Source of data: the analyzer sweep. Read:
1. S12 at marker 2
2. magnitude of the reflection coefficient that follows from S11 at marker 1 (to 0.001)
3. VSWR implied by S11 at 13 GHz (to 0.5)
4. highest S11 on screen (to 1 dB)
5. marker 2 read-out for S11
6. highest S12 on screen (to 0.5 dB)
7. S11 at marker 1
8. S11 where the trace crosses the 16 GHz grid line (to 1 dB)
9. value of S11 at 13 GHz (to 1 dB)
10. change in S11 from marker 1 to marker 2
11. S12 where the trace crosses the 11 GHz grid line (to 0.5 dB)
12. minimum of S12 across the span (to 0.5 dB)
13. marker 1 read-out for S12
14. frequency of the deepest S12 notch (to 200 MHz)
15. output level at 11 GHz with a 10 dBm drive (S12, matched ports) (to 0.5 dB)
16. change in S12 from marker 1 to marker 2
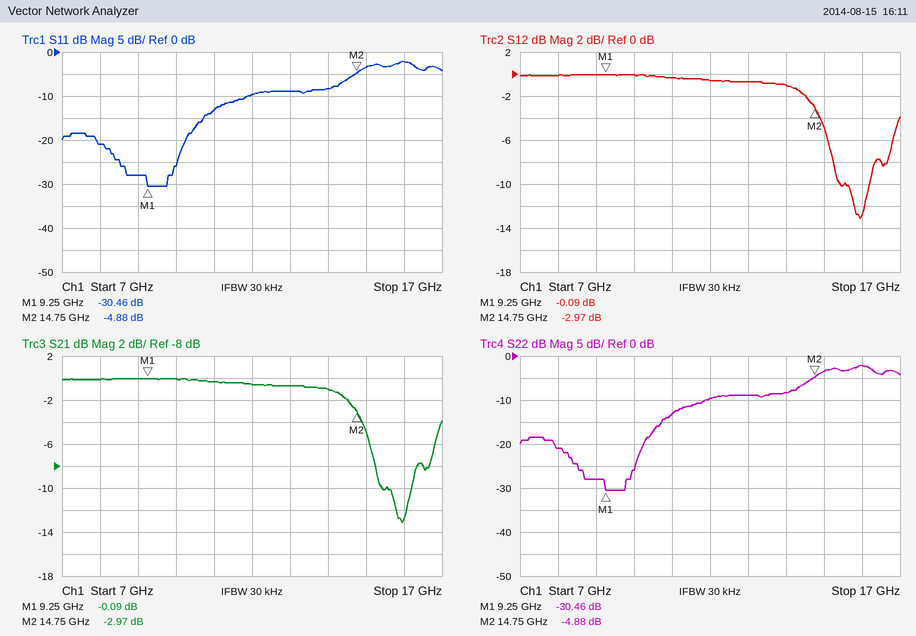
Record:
-2.97 dB
0.030
2.0
-2 dB
-4.88 dB
0.0 dB
-30.46 dB
-2 dB
-9 dB
25.58 dB
-0.5 dB
-13.0 dB
-0.09 dB
16.0 GHz
9.5 dBm
-2.88 dB
